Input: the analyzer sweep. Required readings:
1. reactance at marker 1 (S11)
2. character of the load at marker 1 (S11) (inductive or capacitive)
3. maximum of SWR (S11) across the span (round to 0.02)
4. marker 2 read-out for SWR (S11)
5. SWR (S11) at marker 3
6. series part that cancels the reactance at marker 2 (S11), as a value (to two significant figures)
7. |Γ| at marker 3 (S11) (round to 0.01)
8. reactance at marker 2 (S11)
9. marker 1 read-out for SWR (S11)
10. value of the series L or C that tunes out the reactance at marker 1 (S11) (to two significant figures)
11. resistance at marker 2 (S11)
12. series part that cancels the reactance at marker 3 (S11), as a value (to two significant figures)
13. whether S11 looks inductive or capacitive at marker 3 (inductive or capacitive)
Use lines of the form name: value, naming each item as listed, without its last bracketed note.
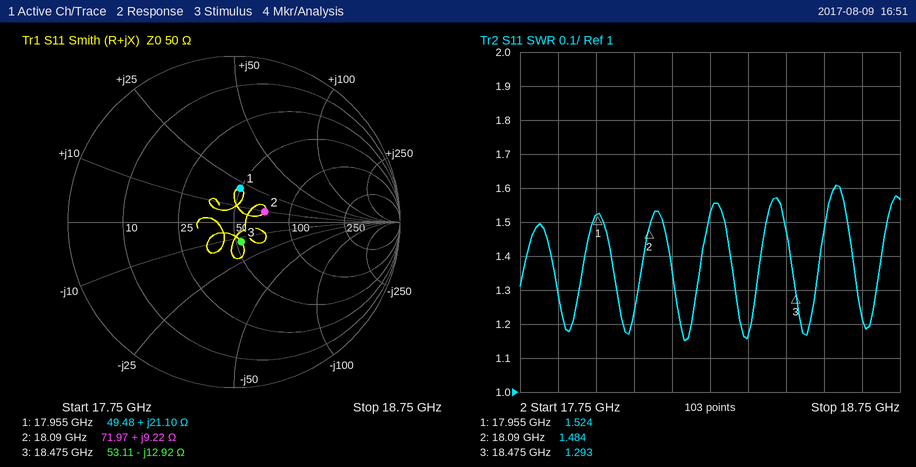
reactance at marker 1: +21.10 Ω
character of the load at marker 1 (S11): inductive
maximum of SWR (S11) across the span: 1.60
marker 2 read-out for SWR: 1.484
SWR (S11) at marker 3: 1.293
series part that cancels the reactance at marker 2 (S11), as a value: 950 fF
|Γ| at marker 3 (S11): 0.13
reactance at marker 2: +9.22 Ω
marker 1 read-out for SWR: 1.524
value of the series L or C that tunes out the reactance at marker 1 (S11): 420 fF
resistance at marker 2: 71.97 Ω
series part that cancels the reactance at marker 3 (S11), as a value: 110 pH
whether S11 looks inductive or capacitive at marker 3: capacitive
